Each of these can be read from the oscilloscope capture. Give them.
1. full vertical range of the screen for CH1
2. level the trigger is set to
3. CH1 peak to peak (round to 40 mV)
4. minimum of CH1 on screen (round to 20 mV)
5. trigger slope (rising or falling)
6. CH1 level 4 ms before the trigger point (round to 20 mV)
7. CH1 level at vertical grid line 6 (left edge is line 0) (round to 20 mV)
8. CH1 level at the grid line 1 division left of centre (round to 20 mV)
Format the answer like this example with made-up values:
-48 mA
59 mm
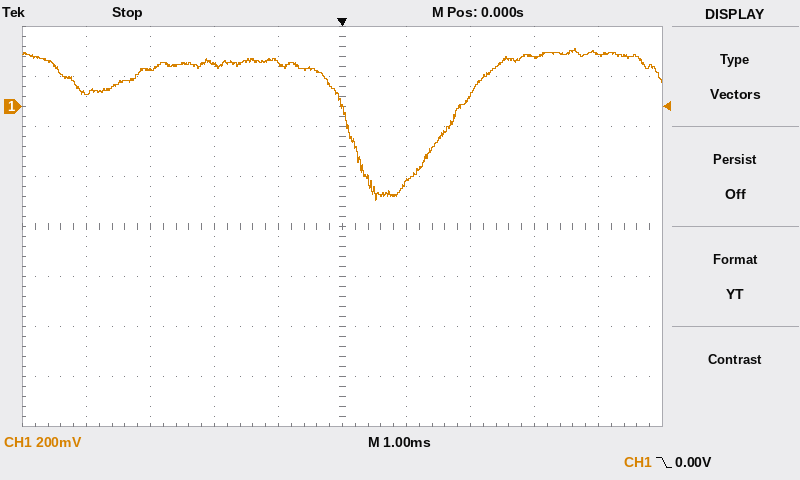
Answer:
1.6 V
0.00 V
600 mV
-380 mV
falling
60 mV
-300 mV
180 mV
